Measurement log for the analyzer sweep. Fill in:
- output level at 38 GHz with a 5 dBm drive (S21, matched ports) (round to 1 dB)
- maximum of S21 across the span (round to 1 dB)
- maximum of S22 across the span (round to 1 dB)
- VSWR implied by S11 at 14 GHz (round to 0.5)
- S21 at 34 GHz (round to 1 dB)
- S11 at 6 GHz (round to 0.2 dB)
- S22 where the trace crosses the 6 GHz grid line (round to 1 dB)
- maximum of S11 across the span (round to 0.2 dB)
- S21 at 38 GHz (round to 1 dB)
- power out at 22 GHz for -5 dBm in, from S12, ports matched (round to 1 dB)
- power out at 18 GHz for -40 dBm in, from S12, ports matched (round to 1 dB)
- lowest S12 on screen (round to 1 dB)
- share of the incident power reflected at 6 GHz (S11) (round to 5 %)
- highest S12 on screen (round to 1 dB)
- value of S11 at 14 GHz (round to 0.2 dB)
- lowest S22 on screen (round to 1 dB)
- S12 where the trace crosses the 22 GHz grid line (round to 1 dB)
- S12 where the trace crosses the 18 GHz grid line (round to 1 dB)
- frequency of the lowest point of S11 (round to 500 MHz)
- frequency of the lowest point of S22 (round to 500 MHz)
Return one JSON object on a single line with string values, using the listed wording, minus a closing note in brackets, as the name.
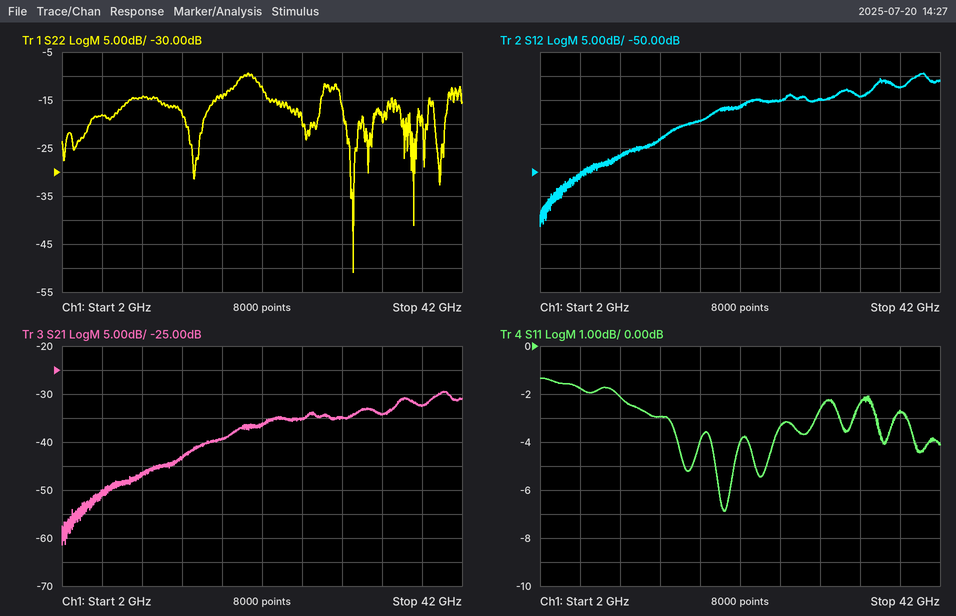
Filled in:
{"output level at 38 GHz with a 5 dBm drive (S21, matched ports)": "-27 dBm", "maximum of S21 across the span": "-29 dB", "maximum of S22 across the span": "-9 dB", "VSWR implied by S11 at 14 GHz": "6.0", "S21 at 34 GHz": "-34 dB", "S11 at 6 GHz": "-1.8 dB", "S22 where the trace crosses the 6 GHz grid line": "-18 dB", "maximum of S11 across the span": "-1.4 dB", "S21 at 38 GHz": "-32 dB", "power out at 22 GHz for -5 dBm in, from S12, ports matched": "-41 dBm", "power out at 18 GHz for -40 dBm in, from S12, ports matched": "-79 dBm", "lowest S12 on screen": "-61 dB", "share of the incident power reflected at 6 GHz (S11)": "65 %", "highest S12 on screen": "-29 dB", "value of S11 at 14 GHz": "-3.0 dB", "lowest S22 on screen": "-51 dB", "S12 where the trace crosses the 22 GHz grid line": "-36 dB", "S12 where the trace crosses the 18 GHz grid line": "-39 dB", "frequency of the lowest point of S11": "20.5 GHz", "frequency of the lowest point of S22": "31.0 GHz"}
